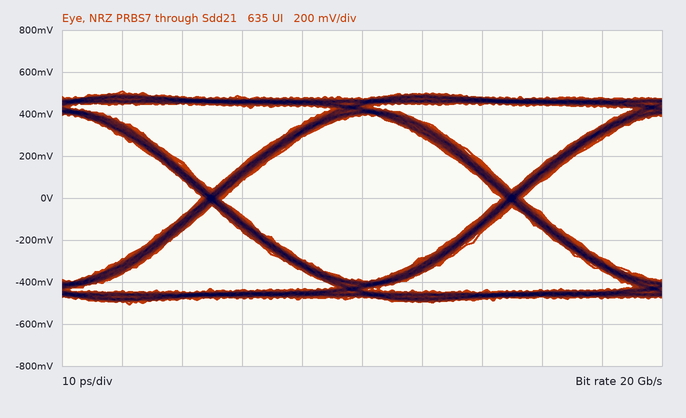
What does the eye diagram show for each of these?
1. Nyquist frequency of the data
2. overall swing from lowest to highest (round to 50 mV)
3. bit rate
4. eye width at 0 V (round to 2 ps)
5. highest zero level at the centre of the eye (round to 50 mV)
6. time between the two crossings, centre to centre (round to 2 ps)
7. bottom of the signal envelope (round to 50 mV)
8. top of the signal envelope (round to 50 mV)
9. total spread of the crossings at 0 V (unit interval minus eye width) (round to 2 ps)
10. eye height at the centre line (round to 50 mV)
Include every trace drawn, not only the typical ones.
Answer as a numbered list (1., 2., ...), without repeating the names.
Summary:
1. 10 GHz
2. 1.00 V
3. 20 Gb/s
4. 46 ps
5. -400 mV
6. 50 ps
7. -500 mV
8. 500 mV
9. 4 ps
10. 800 mV
